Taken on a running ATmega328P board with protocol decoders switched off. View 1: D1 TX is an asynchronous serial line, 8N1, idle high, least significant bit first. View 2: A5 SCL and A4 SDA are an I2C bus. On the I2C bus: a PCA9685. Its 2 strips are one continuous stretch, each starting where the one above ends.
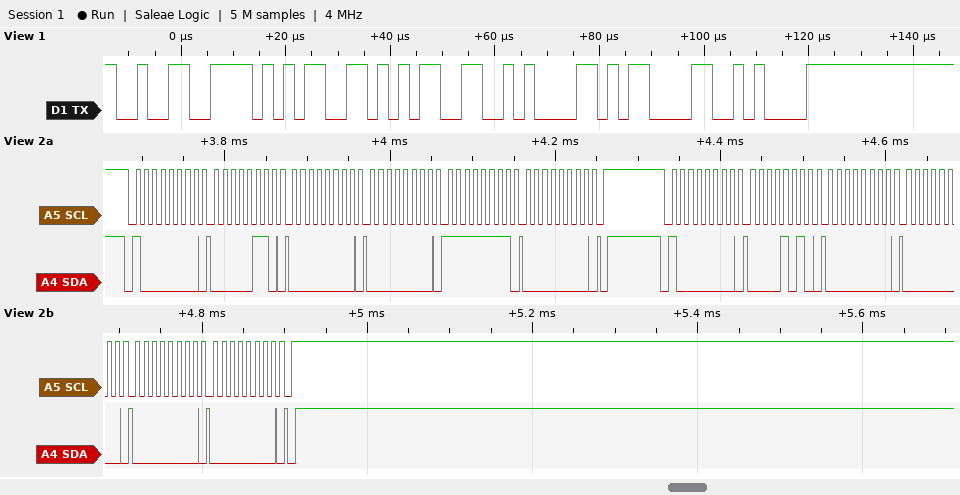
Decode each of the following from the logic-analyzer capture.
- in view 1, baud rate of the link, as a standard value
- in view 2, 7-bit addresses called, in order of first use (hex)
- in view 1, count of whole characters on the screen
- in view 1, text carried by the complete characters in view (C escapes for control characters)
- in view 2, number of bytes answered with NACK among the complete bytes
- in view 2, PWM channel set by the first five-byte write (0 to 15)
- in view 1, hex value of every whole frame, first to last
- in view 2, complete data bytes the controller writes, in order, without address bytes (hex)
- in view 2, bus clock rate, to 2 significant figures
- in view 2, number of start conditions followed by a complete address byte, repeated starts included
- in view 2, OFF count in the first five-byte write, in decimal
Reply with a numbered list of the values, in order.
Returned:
1. 500000 baud
2. 0x40
3. 6
4. "255\n\r\n"
5. 0
6. 0
7. 0x32 0x35 0x35 0x0A 0x0D 0x0A
8. 06 00 00 FF 00 0A 00 00 00 00
9. 100 kHz
10. 2
11. 255
